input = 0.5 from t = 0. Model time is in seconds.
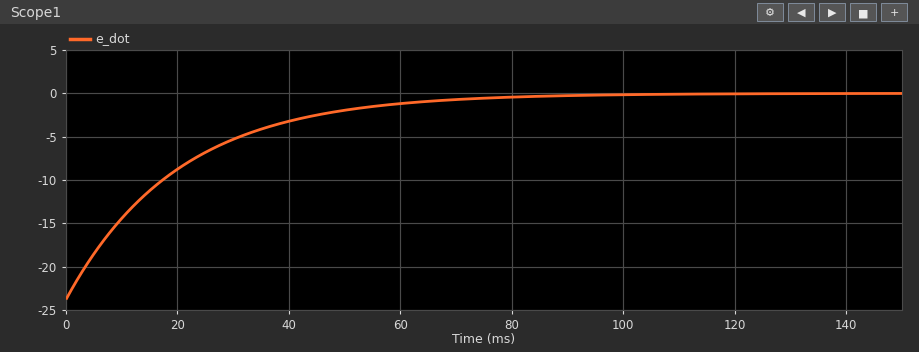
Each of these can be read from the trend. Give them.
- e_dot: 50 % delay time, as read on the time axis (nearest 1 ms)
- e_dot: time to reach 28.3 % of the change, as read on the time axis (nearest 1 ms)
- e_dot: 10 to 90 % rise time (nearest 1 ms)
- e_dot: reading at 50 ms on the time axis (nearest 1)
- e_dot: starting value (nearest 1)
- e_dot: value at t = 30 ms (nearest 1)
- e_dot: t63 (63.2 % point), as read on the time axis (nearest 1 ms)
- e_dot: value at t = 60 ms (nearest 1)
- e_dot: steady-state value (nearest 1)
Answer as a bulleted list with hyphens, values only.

- 14 ms
- 7 ms
- 44 ms
- -2
- -24
- -5
- 20 ms
- -1
- 0
